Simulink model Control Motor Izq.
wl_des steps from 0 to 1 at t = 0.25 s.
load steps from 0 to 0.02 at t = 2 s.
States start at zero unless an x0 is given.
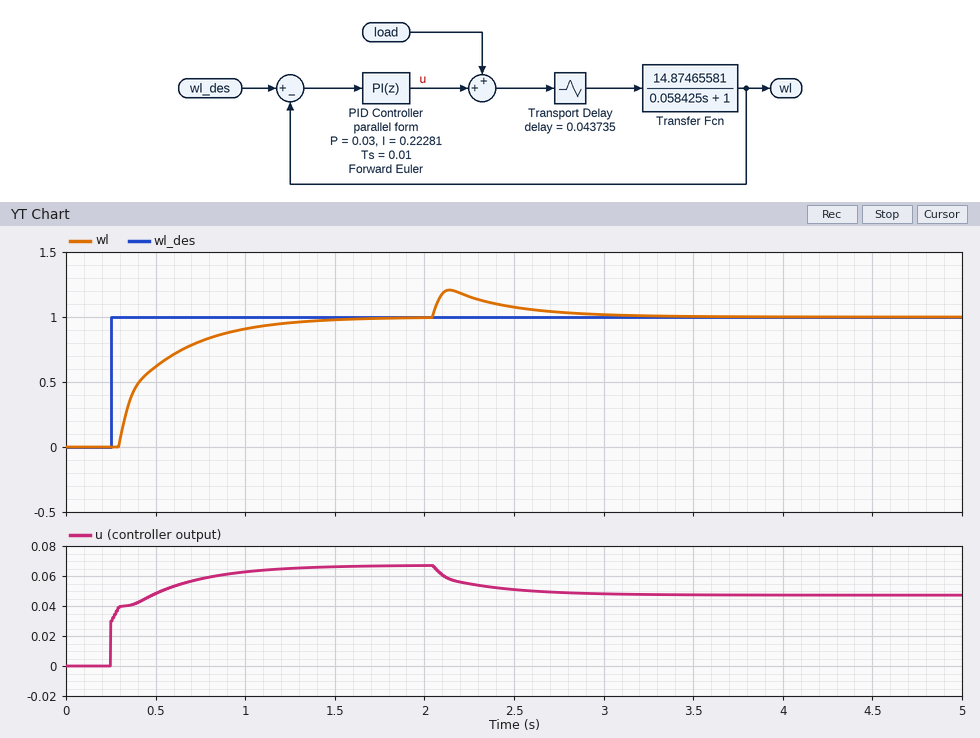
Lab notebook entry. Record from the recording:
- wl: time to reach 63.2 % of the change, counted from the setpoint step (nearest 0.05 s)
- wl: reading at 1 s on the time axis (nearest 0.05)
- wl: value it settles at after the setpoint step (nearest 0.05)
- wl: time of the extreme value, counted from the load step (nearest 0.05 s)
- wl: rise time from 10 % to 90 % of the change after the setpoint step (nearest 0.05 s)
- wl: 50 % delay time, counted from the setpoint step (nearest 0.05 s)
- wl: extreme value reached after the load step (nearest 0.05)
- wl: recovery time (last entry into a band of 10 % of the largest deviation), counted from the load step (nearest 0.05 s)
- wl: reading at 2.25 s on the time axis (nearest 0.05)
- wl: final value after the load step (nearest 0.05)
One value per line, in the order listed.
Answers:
0.25 s
0.90
1.00
0.15 s
0.65 s
0.15 s
1.20
0.95 s
1.15
1.00
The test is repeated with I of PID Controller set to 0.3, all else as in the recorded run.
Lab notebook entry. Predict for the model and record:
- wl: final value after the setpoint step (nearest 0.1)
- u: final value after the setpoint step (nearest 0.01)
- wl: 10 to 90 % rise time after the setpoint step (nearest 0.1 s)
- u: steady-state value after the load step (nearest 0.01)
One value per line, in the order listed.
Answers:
1.0
0.07
0.4 s
0.05
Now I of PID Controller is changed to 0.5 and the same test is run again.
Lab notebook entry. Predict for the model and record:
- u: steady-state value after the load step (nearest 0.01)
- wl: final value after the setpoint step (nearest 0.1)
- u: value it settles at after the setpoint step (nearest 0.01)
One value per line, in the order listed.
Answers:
0.05
1.0
0.07
